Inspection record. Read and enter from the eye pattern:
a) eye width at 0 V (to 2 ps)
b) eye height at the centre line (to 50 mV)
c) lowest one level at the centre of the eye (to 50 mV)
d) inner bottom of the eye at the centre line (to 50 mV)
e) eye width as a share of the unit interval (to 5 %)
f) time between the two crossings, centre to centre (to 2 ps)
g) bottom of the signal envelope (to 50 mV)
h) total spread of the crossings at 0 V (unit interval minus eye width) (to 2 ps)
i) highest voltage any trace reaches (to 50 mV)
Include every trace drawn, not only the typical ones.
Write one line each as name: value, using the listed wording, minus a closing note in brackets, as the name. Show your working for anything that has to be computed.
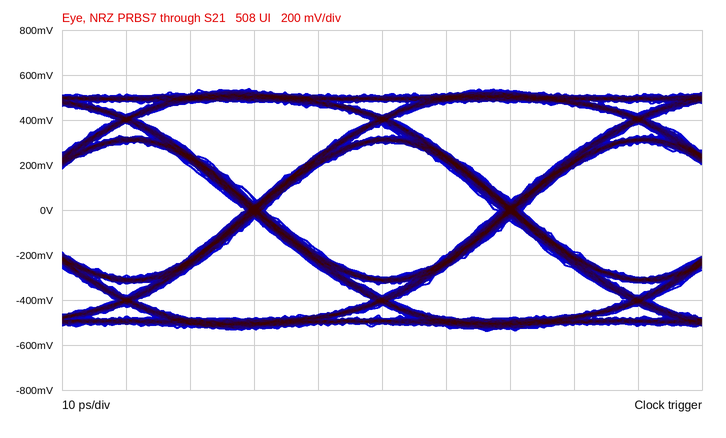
eye width at 0 V: 36 ps
eye height at the centre line: 600 mV
lowest one level at the centre of the eye: 300 mV
inner bottom of the eye at the centre line: -300 mV
eye width as a share of the unit interval: 36 ps / 40 ps ≈ 90 %
time between the two crossings, centre to centre: 40 ps
bottom of the signal envelope: -550 mV
total spread of the crossings at 0 V (unit interval minus eye width): 4 ps
highest voltage any trace reaches: 550 mV
